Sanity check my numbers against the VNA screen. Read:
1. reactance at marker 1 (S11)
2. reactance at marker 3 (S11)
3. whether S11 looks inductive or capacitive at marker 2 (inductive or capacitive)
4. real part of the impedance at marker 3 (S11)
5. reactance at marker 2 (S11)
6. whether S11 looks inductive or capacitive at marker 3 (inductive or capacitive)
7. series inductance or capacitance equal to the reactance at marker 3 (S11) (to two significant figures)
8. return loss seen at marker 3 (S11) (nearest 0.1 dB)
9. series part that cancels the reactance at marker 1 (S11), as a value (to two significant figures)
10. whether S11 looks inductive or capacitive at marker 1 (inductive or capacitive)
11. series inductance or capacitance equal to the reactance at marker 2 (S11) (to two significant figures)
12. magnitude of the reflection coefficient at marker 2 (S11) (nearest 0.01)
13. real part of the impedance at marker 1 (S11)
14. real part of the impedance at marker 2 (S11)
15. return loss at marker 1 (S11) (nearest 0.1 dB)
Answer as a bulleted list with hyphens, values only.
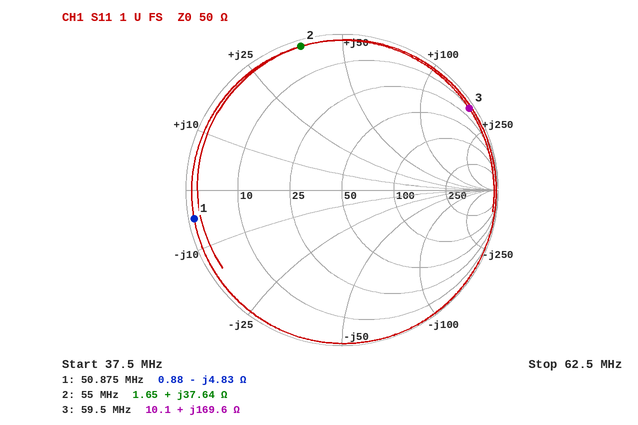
- -4.83 Ω
- +169.6 Ω
- inductive
- 10.1 Ω
- +37.64 Ω
- inductive
- 450 nH
- 0.3 dB
- 15 nH
- capacitive
- 110 nH
- 0.96
- 0.88 Ω
- 1.65 Ω
- 0.3 dB
